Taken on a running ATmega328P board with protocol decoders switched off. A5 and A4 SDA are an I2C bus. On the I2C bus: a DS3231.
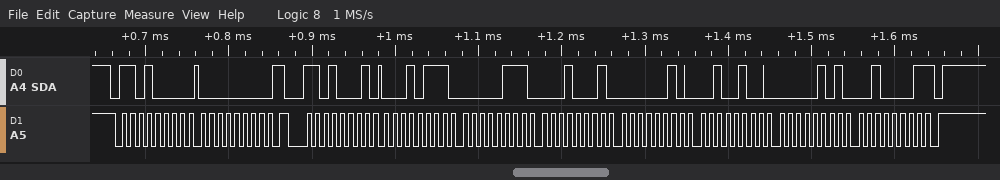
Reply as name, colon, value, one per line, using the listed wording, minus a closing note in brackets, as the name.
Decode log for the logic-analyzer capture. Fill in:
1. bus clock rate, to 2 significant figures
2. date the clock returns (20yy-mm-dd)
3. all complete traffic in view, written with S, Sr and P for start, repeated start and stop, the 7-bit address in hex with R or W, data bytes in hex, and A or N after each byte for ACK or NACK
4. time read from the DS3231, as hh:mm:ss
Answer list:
bus clock rate, to 2 significant figures: 100 kHz
date the clock returns: 2021-05-24
all complete traffic in view, written with S, Sr and P for start, repeated start and stop, the 7-bit address in hex with R or W, data bytes in hex, and A or N after each byte for ACK or NACK: S 68W A 00 A Sr 68R A 17 A 07 A 11 A 02 A 24 A 05 A 21 N P
time read from the DS3231, as hh:mm:ss: 11:07:17
